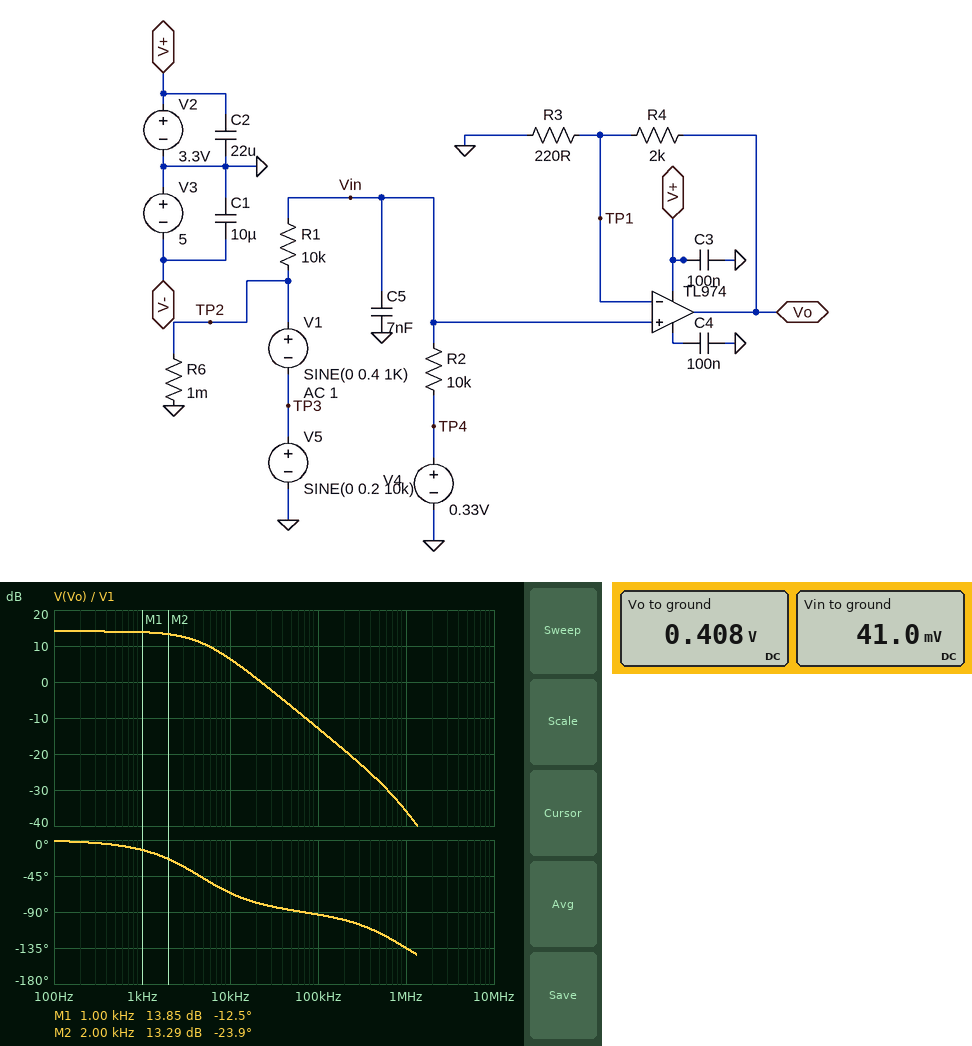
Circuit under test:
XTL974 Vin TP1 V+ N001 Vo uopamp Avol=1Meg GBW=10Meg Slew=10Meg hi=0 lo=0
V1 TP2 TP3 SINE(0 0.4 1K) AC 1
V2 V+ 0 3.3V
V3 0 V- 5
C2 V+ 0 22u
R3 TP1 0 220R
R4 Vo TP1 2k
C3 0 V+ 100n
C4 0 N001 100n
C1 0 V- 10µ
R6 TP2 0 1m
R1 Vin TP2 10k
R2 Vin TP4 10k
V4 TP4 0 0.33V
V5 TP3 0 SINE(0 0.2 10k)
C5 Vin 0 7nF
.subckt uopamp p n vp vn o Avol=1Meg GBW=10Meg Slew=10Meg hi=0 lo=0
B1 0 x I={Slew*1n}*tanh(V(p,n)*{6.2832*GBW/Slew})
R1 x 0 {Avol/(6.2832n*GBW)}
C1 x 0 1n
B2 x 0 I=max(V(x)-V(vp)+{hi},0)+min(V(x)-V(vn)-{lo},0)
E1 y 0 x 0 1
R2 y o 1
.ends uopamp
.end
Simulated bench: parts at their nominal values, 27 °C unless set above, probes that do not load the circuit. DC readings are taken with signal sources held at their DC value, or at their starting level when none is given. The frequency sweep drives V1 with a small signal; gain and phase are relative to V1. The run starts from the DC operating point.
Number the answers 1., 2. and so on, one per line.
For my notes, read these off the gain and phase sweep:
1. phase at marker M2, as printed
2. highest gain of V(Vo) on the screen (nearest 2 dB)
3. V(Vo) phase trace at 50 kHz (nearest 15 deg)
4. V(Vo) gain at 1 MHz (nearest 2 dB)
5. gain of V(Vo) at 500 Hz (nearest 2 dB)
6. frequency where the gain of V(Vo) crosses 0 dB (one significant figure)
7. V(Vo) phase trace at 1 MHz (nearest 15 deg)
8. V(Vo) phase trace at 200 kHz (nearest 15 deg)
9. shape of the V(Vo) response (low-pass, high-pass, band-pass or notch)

1. -23.9 deg
2. 14 dB
3. -90 deg
4. -36 dB
5. 14 dB
6. 20 kHz
7. -135 deg
8. -105 deg
9. low-pass
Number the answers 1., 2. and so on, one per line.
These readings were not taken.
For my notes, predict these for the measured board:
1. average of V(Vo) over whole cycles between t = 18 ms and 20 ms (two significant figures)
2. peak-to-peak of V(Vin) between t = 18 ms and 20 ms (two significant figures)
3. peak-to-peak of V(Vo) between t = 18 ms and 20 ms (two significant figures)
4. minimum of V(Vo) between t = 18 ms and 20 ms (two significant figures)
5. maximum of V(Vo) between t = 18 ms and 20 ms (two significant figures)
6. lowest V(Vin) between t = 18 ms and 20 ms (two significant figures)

1. 1.7 V
2. 470 mV
3. 3.3 V
4. -4.2 mV
5. 3.3 V
6. -71 mV
